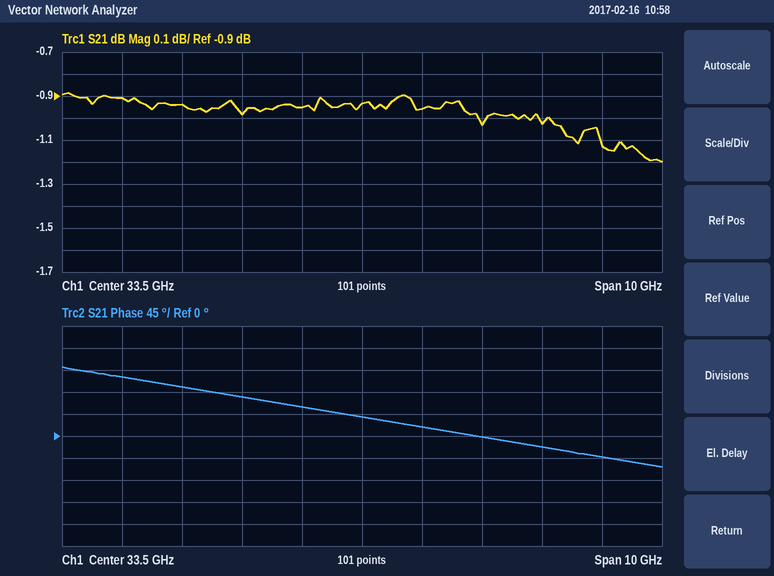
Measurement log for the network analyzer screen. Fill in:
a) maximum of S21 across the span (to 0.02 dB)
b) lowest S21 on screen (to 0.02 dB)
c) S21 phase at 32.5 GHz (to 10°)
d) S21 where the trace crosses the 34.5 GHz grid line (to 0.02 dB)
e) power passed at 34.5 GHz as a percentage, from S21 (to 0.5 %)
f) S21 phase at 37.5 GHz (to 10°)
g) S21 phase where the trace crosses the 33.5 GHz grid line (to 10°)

-0.88 dB
-1.20 dB
60°
-0.96 dB
80.0 %
-40°
40°
